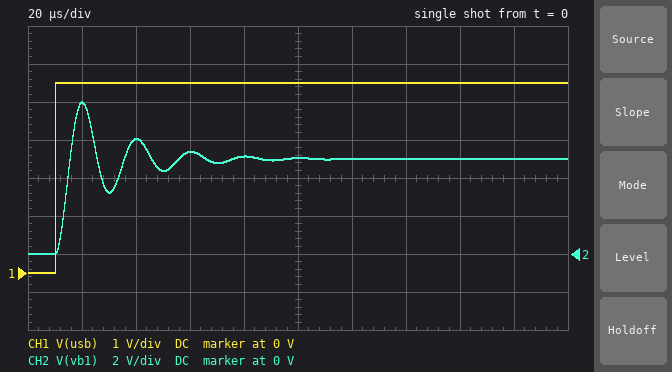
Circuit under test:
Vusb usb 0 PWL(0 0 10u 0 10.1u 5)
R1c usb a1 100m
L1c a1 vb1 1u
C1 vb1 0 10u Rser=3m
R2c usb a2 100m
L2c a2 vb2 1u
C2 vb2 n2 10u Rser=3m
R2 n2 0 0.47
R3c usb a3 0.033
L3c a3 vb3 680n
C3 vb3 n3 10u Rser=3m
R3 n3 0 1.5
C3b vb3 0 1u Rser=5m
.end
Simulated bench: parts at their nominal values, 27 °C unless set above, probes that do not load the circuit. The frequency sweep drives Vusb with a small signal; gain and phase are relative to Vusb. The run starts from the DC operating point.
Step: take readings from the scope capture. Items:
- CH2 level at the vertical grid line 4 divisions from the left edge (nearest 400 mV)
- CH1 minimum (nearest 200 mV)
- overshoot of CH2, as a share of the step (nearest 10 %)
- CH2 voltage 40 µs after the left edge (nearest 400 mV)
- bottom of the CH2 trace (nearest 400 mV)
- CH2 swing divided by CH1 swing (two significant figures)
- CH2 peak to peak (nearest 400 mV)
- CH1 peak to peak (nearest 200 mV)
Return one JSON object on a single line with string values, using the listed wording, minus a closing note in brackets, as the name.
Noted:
{"CH2 level at the vertical grid line 4 divisions from the left edge": "5.2 V", "CH1 minimum": "0 V", "overshoot of CH2, as a share of the step": "60 %", "CH2 voltage 40 µs after the left edge": "6.0 V", "bottom of the CH2 trace": "0 V", "CH2 swing divided by CH1 swing": "1.6", "CH2 peak to peak": "8.0 V", "CH1 peak to peak": "5.0 V"}
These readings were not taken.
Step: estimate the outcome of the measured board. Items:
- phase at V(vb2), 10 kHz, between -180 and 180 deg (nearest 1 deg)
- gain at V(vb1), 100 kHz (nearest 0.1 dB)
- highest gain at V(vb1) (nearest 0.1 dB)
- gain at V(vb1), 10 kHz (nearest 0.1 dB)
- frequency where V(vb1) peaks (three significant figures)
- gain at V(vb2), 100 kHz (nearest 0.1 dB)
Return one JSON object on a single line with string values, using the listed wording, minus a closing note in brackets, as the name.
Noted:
{"phase at V(vb2), 10 kHz, between -180 and 180 deg": "-4 deg", "gain at V(vb1), 100 kHz": "-9.6 dB", "highest gain at V(vb1)": "9.9 dB", "gain at V(vb1), 10 kHz": "0.3 dB", "frequency where V(vb1) peaks": "49.0 kHz", "gain at V(vb2), 100 kHz": "-3.4 dB"}
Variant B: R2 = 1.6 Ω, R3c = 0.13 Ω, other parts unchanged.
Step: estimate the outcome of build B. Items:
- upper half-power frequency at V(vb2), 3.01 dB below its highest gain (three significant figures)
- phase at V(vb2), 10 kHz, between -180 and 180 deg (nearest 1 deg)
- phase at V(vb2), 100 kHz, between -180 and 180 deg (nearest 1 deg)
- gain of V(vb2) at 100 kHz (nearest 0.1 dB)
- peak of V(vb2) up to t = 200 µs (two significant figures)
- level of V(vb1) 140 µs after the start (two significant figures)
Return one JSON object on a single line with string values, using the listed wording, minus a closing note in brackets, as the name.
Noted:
{"upper half-power frequency at V(vb2), 3.01 dB below its highest gain": "249 kHz", "phase at V(vb2), 10 kHz, between -180 and 180 deg": "-3 deg", "phase at V(vb2), 100 kHz, between -180 and 180 deg": "-21 deg", "gain of V(vb2) at 100 kHz": "-0.8 dB", "peak of V(vb2) up to t = 200 µs": "5.0 V", "level of V(vb1) 140 µs after the start": "5.0 V"}
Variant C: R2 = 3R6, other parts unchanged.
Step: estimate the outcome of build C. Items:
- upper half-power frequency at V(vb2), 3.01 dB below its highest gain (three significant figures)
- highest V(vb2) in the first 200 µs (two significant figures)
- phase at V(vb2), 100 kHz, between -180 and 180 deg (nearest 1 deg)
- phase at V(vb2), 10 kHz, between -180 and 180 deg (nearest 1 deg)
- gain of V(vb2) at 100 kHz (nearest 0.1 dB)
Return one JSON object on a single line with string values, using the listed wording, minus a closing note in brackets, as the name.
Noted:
{"upper half-power frequency at V(vb2), 3.01 dB below its highest gain": "562 kHz", "highest V(vb2) in the first 200 µs": "5.0 V", "phase at V(vb2), 100 kHz, between -180 and 180 deg": "-10 deg", "phase at V(vb2), 10 kHz, between -180 and 180 deg": "-1 deg", "gain of V(vb2) at 100 kHz": "-0.3 dB"}
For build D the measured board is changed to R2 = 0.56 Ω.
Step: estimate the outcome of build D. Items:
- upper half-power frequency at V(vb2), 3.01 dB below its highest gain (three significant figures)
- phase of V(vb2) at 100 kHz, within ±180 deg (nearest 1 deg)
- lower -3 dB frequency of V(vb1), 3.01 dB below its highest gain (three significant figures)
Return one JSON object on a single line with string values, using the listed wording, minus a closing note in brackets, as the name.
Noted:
{"upper half-power frequency at V(vb2), 3.01 dB below its highest gain": "96.9 kHz", "phase of V(vb2) at 100 kHz, within ±180 deg": "-51 deg", "lower -3 dB frequency of V(vb1), 3.01 dB below its highest gain": "39.8 kHz"}
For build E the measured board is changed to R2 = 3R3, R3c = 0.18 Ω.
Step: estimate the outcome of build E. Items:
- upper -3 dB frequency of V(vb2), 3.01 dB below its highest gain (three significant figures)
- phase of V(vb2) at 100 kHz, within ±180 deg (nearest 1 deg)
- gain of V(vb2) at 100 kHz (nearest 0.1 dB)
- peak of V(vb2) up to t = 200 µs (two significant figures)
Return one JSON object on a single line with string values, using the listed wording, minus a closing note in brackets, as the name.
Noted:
{"upper -3 dB frequency of V(vb2), 3.01 dB below its highest gain": "514 kHz", "phase of V(vb2) at 100 kHz, within ±180 deg": "-11 deg", "gain of V(vb2) at 100 kHz": "-0.3 dB", "peak of V(vb2) up to t = 200 µs": "5.0 V"}
